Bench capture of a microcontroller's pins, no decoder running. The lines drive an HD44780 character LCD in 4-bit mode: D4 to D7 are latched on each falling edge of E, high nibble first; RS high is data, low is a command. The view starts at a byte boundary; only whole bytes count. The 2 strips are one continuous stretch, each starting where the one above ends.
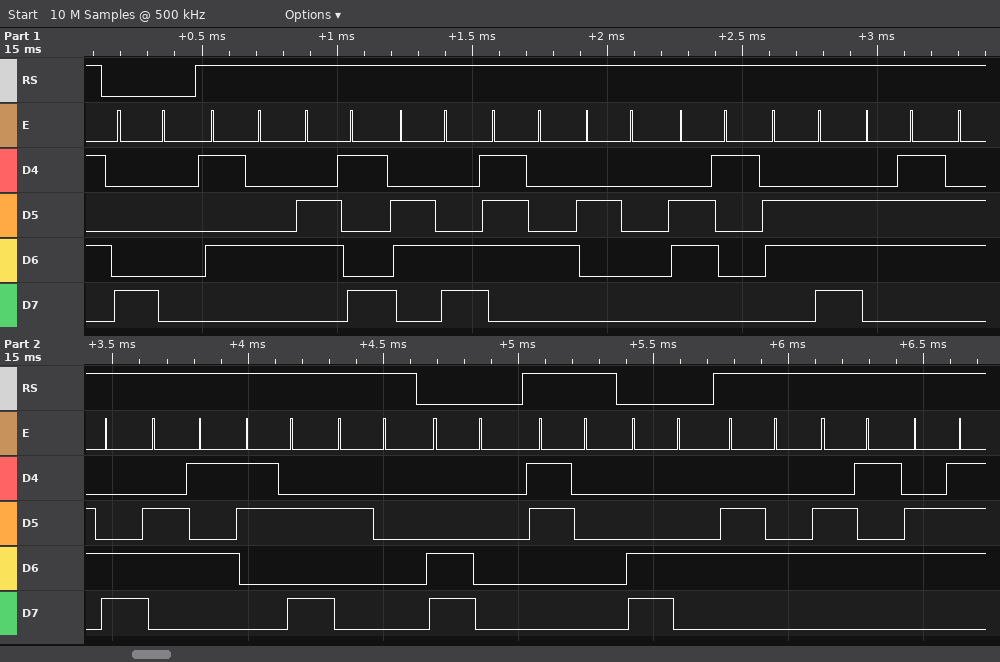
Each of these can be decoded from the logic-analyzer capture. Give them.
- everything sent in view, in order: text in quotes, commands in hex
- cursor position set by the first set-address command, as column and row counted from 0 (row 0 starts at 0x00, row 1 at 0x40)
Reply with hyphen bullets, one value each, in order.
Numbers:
- 0x80 "Tilt angle: " 0xC0 "0" 0xC4 "deg"
- column 0, row 0
